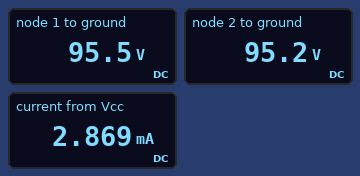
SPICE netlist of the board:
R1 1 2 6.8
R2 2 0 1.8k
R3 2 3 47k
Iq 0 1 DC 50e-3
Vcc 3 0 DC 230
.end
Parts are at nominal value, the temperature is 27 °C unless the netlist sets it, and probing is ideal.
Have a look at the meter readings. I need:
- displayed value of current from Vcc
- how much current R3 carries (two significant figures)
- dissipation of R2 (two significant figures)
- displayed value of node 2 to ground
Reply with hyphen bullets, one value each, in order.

- 2.869 mA
- 2.9 mA
- 5.0 W
- 95.2 V
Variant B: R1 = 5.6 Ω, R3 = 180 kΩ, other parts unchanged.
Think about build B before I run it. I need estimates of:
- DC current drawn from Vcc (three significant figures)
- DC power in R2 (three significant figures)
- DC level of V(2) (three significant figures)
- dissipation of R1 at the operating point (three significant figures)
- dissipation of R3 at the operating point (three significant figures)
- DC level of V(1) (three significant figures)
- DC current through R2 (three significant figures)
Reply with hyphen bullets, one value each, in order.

- 770 µA
- 4.64 W
- 91.4 V
- 14.0 mW
- 107 mW
- 91.7 V
- 50.8 mA
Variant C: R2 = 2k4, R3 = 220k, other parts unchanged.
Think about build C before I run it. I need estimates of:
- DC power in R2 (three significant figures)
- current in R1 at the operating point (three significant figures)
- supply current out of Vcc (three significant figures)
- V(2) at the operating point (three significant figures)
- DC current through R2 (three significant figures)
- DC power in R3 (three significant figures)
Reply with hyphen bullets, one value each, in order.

- 6.12 W
- 50.0 mA
- 495 µA
- 121 V
- 50.5 mA
- 53.8 mW
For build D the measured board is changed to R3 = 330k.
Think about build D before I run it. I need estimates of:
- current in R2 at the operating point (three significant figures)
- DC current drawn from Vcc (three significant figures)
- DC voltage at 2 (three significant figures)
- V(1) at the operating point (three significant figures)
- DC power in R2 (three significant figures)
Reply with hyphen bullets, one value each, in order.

- 50.4 mA
- 422 µA
- 90.8 V
- 91.1 V
- 4.58 W
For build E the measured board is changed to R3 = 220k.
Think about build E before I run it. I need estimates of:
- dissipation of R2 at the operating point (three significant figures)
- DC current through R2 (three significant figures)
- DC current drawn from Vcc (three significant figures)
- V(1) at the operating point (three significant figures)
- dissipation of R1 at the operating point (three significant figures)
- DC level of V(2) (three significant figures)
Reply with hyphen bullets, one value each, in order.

- 4.61 W
- 50.6 mA
- 631 µA
- 91.5 V
- 17.0 mW
- 91.1 V
